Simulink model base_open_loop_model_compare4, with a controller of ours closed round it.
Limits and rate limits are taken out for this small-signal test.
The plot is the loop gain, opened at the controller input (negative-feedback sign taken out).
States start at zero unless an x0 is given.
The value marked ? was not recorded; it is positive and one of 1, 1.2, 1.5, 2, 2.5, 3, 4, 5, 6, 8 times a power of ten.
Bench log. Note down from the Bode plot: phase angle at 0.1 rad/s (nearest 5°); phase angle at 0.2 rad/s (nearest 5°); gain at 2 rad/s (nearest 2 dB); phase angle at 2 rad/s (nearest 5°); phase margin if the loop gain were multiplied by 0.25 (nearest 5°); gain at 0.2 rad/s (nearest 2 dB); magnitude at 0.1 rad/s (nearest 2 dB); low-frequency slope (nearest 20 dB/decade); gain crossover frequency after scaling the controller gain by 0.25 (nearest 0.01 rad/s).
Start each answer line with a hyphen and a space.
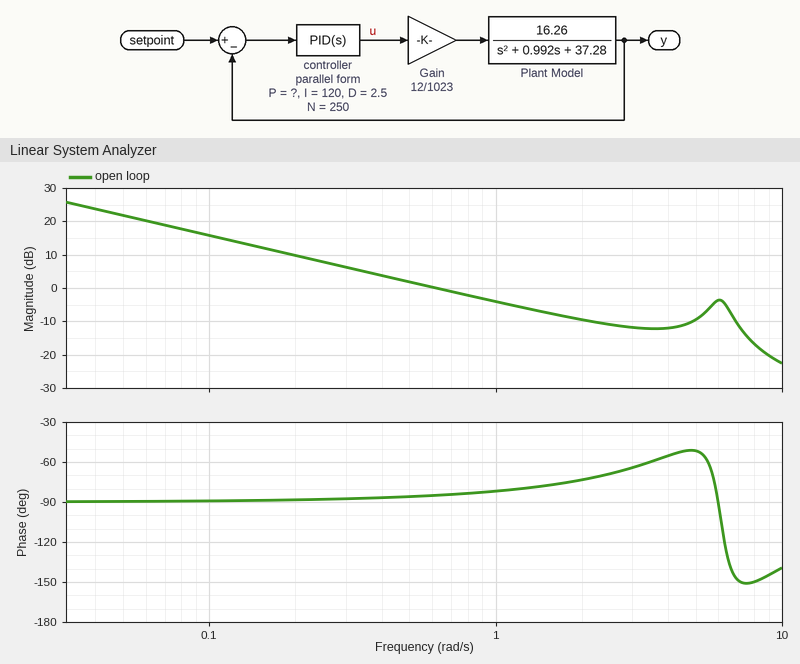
- -90°
- -90°
- -10 dB
- -75°
- 90°
- 10 dB
- 16 dB
- -20 dB/decade
- 0.15 rad/s
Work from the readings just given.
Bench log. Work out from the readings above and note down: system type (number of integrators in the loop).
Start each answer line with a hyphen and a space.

- 1
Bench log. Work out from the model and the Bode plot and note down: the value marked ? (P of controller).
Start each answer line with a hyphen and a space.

- 20
